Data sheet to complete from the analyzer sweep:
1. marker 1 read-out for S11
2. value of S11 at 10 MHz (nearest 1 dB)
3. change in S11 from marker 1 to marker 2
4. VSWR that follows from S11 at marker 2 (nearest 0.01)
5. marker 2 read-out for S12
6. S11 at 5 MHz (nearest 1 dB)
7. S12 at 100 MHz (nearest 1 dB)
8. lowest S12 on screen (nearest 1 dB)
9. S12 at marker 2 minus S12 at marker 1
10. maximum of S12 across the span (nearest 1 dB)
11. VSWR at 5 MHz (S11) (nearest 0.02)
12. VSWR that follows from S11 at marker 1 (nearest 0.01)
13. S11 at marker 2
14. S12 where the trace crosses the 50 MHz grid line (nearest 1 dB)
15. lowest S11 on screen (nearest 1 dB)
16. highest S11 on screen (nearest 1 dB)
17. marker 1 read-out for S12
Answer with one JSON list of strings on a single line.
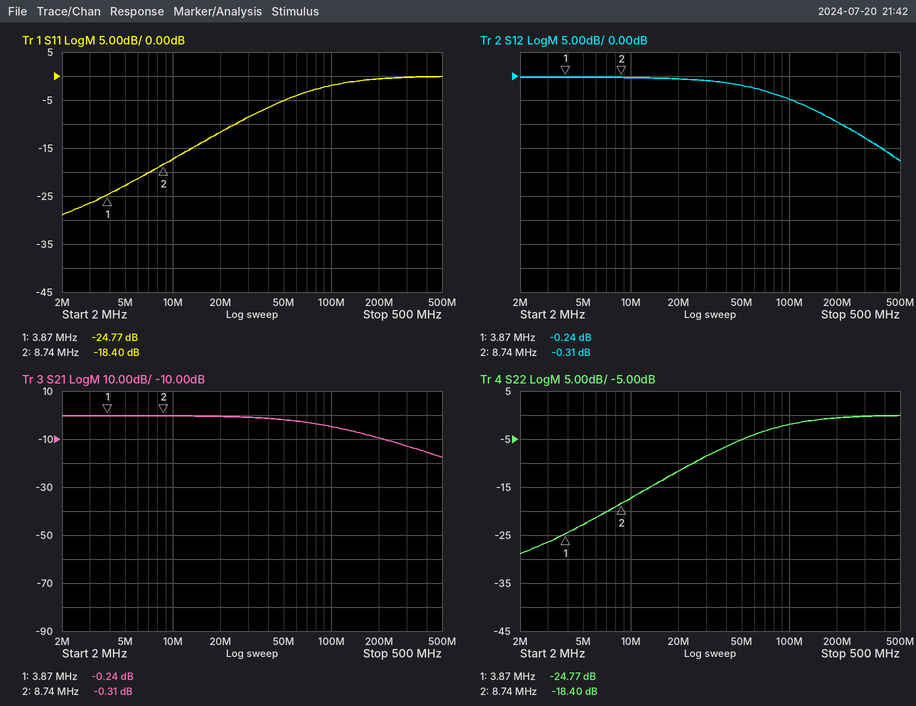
["-24.77 dB", "-17 dB", "6.37 dB", "1.27", "-0.31 dB", "-23 dB", "-5 dB", "-18 dB", "-0.07 dB", "0 dB", "1.16", "1.12", "-18.40 dB", "-2 dB", "-29 dB", "0 dB", "-0.24 dB"]
